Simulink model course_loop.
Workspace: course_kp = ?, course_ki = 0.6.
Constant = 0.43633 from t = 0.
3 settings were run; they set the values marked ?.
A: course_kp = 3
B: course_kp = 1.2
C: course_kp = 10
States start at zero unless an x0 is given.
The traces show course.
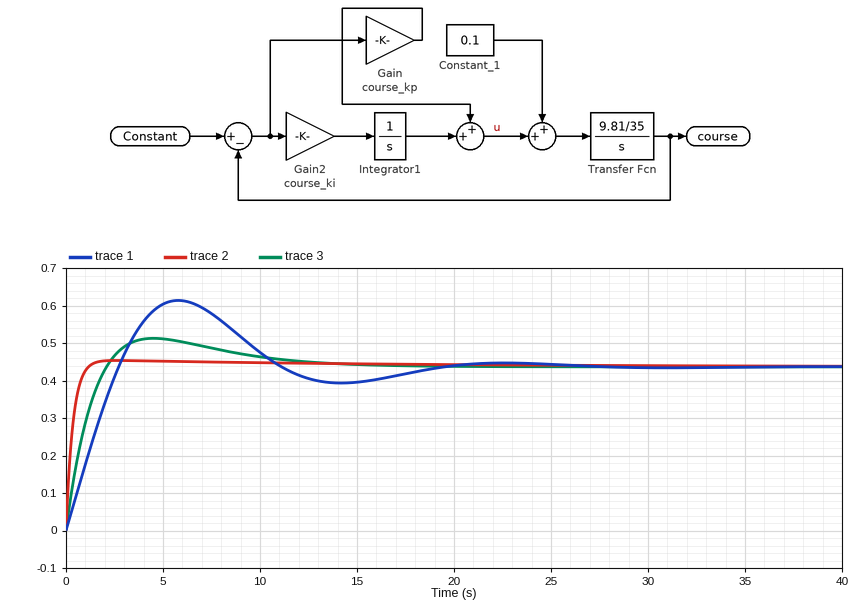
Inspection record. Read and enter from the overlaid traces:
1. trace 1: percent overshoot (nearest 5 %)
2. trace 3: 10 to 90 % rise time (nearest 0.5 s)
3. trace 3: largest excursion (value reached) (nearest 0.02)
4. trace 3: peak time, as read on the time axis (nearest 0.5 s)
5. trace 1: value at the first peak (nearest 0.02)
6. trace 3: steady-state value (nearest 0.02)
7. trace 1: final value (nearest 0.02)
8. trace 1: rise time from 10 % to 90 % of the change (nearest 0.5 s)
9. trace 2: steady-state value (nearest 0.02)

40 %
1.5 s
0.52
4.5 s
0.62
0.44
0.44
2.0 s
0.44
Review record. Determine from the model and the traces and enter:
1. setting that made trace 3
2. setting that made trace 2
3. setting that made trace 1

A
C
B
